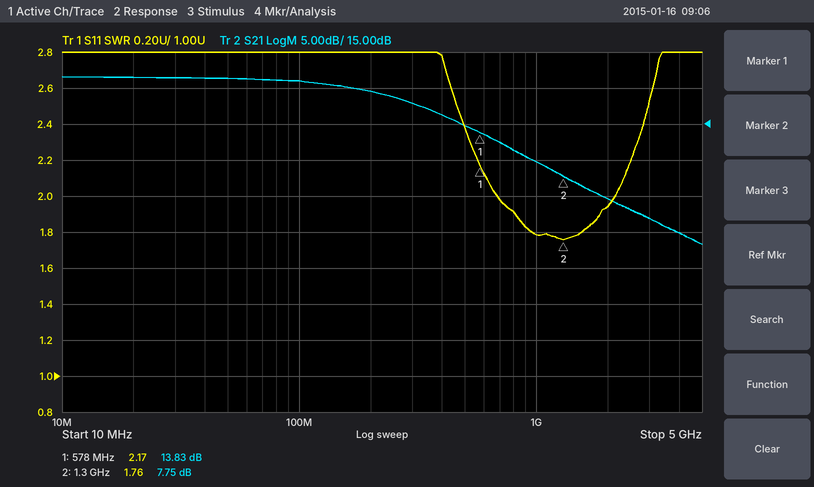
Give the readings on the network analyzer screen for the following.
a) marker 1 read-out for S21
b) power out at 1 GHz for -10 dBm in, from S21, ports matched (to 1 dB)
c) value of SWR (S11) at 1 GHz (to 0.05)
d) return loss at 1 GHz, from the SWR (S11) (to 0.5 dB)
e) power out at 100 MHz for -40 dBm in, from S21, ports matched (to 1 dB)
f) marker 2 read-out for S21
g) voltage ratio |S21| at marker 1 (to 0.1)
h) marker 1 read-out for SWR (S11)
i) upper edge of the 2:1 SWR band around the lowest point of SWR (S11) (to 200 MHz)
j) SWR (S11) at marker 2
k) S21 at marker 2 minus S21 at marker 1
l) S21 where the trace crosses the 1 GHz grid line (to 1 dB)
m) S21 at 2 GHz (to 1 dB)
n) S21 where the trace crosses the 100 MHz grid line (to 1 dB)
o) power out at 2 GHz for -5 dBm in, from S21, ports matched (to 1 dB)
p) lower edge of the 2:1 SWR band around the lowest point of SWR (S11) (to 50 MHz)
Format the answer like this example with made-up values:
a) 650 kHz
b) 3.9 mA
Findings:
a) 13.83 dB
b) 0 dBm
c) 1.80
d) 11.0 dB
e) -19 dBm
f) 7.75 dB
g) 4.9
h) 2.17
i) 2.2 GHz
j) 1.76
k) -6.08 dB
l) 10 dB
m) 5 dB
n) 21 dB
o) 0 dBm
p) 700 MHz
